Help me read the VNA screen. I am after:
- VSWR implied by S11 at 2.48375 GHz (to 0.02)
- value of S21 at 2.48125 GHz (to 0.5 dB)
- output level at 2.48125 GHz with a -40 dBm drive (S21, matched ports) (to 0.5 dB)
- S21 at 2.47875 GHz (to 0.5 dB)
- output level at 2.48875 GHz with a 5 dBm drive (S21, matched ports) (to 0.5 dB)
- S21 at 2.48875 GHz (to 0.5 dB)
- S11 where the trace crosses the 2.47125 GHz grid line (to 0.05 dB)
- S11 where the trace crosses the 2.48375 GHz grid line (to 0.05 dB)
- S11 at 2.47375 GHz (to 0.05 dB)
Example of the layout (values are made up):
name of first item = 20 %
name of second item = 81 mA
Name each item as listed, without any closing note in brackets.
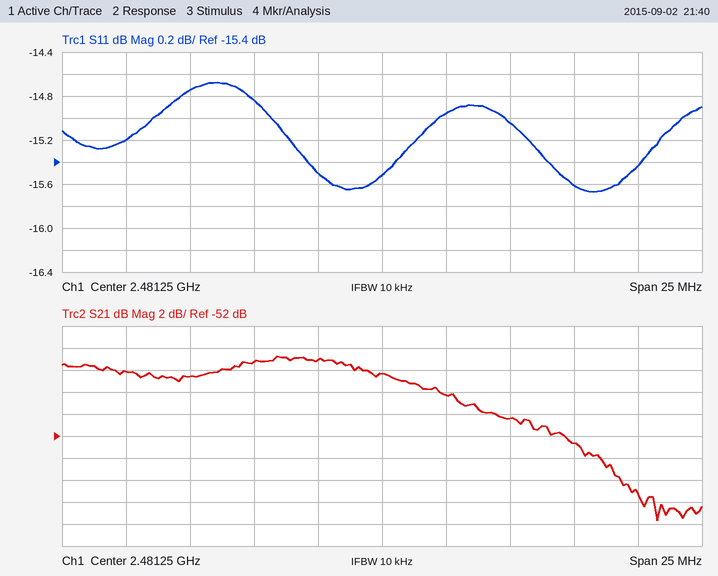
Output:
VSWR implied by S11 at 2.48375 GHz = 1.44
value of S21 at 2.48125 GHz = -46.5 dB
output level at 2.48125 GHz with a -40 dBm drive (S21, matched ports) = -86.5 dBm
S21 at 2.47875 GHz = -45.0 dB
output level at 2.48875 GHz with a 5 dBm drive (S21, matched ports) = -47.5 dBm
S21 at 2.48875 GHz = -52.5 dB
S11 where the trace crosses the 2.47125 GHz grid line = -15.20 dB
S11 where the trace crosses the 2.48375 GHz grid line = -14.95 dB
S11 at 2.47375 GHz = -14.75 dB
